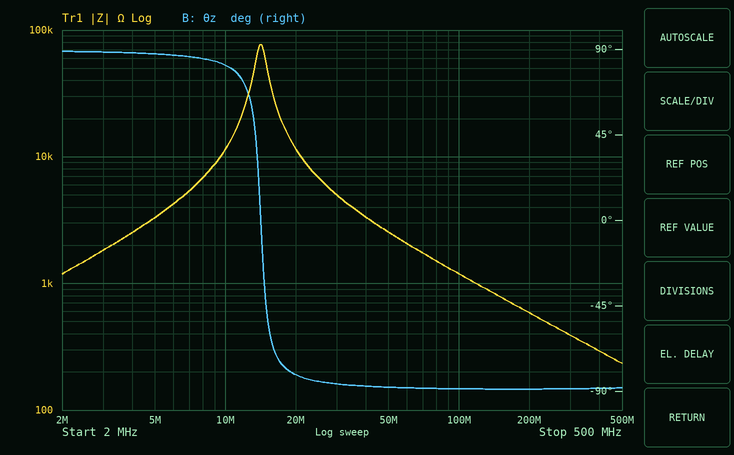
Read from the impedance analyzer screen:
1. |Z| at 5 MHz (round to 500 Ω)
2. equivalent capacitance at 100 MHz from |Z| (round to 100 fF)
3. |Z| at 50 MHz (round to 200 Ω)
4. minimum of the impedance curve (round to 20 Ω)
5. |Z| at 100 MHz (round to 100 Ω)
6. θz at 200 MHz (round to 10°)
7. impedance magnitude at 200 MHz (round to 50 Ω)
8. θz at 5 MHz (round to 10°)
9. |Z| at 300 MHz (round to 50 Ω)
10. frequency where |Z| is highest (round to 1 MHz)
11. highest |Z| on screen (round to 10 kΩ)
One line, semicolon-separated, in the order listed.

3.5 kΩ; 1.3 pF; 2.6 kΩ; 240 Ω; 1.2 kΩ; -90°; 600 Ω; 90°; 400 Ω; 14 MHz; 80 kΩ
